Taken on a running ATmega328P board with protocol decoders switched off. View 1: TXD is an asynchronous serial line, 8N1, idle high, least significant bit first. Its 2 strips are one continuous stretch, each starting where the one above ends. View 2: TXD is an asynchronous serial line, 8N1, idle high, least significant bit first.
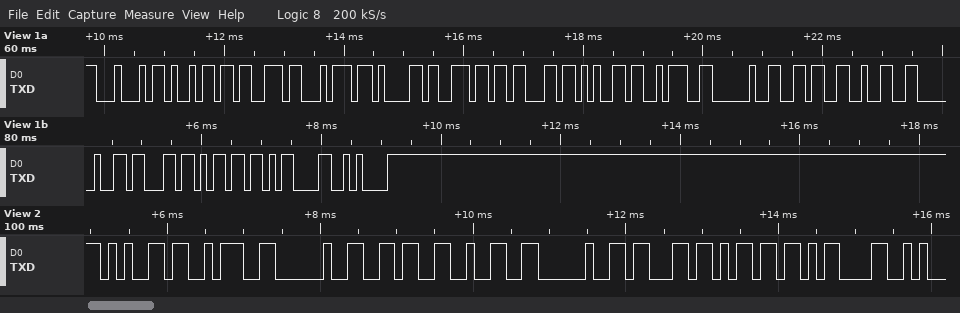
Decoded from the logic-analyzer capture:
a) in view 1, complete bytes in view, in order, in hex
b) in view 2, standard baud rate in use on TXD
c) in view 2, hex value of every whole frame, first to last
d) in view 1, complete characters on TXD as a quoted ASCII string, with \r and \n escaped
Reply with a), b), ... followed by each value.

a) 44 69 73 74 61 6E 63 65 3A 20 36 32 20 63 6D 0D 0A
b) 9600 baud
c) 65 3A 20 36 32 20 63 6D 0D
d) "Distance: 62 cm\r\n"
